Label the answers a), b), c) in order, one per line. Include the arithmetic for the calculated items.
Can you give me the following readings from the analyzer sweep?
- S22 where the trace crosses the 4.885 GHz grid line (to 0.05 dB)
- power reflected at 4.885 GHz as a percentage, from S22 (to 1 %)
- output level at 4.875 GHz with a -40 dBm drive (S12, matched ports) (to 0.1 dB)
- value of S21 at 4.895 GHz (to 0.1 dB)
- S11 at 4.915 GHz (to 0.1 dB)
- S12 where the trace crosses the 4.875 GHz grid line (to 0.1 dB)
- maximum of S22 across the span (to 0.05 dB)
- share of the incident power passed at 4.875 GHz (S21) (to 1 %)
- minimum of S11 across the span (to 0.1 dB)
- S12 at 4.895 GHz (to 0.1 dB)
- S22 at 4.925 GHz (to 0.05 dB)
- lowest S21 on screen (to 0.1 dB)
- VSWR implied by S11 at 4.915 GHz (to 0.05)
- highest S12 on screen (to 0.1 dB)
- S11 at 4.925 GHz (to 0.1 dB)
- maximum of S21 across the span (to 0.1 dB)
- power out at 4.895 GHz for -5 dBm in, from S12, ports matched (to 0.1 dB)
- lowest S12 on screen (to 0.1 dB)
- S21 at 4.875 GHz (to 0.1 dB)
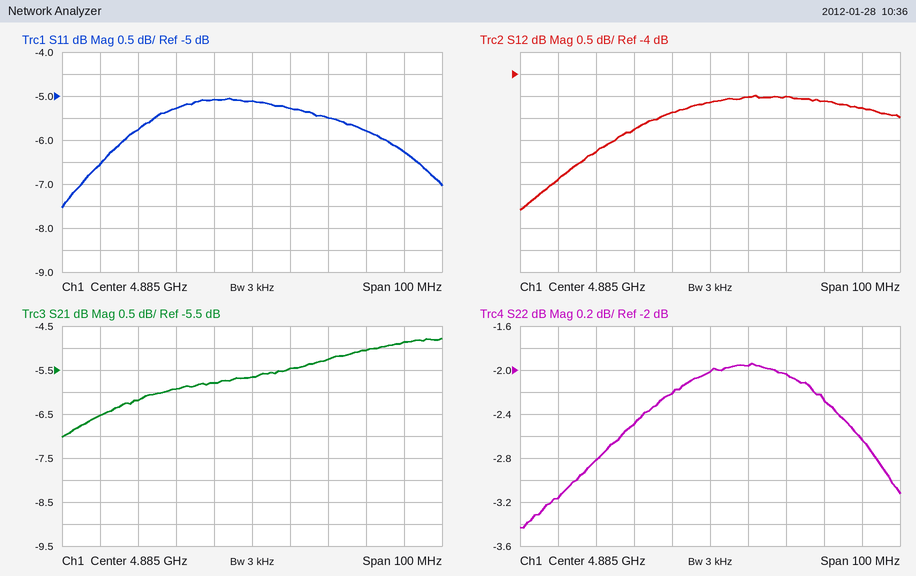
a) -2.00 dB
b) 10^(-2/10) ≈ 63 %
c) -40 dBm + (-4.9 dB) = -44.9 dBm
d) -5.5 dB
e) -5.8 dB
f) -4.9 dB
g) -1.95 dB
h) 10^(-5.8/10) ≈ 26 %
i) -7.5 dB
j) -4.5 dB
k) -2.65 dB
l) -7.0 dB
m) |Γ| = 10^(-5.8/20) = 0.5129; VSWR = (1 + 0.5129)/(1 − 0.5129) ≈ 3.11, so 3.10 to the nearest 0.05
n) -4.5 dB
o) -6.3 dB
p) -4.8 dB
q) -5 dBm + (-4.5 dB) = -9.5 dBm
r) -7.1 dB
s) -5.8 dB
